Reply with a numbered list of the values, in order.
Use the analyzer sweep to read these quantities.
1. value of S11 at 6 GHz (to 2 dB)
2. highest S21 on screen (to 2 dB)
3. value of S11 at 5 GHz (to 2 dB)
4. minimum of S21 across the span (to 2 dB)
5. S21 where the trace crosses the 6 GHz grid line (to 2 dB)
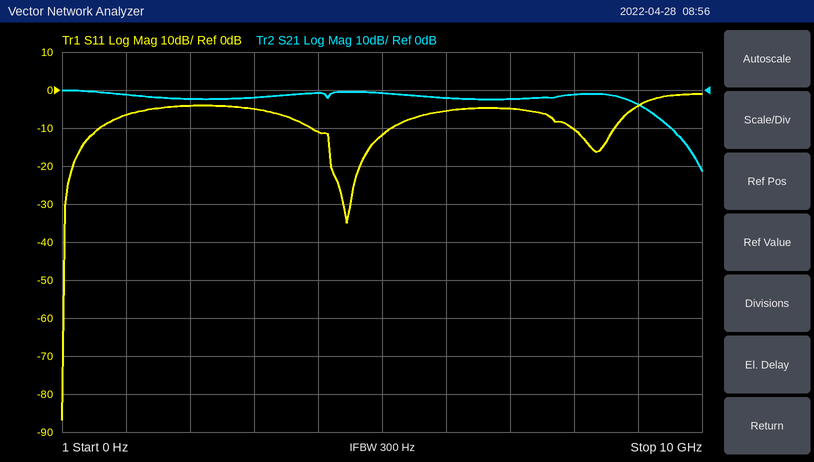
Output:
1. -6 dB
2. 0 dB
3. -12 dB
4. -22 dB
5. -2 dB
